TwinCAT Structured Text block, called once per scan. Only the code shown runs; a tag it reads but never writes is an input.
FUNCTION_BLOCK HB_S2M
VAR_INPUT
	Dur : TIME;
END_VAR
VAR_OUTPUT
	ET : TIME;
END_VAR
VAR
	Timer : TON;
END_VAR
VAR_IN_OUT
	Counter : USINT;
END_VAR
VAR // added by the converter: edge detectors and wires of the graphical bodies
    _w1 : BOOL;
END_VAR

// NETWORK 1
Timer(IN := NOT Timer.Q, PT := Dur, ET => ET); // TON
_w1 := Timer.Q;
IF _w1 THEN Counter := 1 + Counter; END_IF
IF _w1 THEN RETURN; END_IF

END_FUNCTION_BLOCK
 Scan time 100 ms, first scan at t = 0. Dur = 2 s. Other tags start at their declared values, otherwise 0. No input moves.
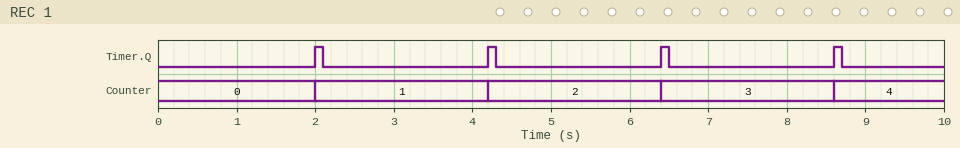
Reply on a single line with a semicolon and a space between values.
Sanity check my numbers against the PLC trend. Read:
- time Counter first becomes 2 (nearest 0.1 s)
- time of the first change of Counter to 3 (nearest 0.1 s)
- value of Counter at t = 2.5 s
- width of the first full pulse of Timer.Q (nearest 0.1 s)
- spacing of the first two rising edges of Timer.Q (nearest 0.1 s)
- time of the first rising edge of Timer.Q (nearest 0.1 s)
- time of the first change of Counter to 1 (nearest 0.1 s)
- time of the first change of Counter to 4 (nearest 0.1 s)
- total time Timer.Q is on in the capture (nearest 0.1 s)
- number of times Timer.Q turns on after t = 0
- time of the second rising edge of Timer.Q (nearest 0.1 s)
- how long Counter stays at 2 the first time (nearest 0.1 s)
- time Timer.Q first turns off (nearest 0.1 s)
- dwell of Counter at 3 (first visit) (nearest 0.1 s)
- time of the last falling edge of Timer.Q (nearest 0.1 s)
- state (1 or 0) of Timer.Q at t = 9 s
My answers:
4.2 s; 6.4 s; 1; 0.1 s; 2.2 s; 2.0 s; 2.0 s; 8.6 s; 0.4 s; 4; 4.2 s; 2.2 s; 2.1 s; 2.2 s; 8.7 s; 0
